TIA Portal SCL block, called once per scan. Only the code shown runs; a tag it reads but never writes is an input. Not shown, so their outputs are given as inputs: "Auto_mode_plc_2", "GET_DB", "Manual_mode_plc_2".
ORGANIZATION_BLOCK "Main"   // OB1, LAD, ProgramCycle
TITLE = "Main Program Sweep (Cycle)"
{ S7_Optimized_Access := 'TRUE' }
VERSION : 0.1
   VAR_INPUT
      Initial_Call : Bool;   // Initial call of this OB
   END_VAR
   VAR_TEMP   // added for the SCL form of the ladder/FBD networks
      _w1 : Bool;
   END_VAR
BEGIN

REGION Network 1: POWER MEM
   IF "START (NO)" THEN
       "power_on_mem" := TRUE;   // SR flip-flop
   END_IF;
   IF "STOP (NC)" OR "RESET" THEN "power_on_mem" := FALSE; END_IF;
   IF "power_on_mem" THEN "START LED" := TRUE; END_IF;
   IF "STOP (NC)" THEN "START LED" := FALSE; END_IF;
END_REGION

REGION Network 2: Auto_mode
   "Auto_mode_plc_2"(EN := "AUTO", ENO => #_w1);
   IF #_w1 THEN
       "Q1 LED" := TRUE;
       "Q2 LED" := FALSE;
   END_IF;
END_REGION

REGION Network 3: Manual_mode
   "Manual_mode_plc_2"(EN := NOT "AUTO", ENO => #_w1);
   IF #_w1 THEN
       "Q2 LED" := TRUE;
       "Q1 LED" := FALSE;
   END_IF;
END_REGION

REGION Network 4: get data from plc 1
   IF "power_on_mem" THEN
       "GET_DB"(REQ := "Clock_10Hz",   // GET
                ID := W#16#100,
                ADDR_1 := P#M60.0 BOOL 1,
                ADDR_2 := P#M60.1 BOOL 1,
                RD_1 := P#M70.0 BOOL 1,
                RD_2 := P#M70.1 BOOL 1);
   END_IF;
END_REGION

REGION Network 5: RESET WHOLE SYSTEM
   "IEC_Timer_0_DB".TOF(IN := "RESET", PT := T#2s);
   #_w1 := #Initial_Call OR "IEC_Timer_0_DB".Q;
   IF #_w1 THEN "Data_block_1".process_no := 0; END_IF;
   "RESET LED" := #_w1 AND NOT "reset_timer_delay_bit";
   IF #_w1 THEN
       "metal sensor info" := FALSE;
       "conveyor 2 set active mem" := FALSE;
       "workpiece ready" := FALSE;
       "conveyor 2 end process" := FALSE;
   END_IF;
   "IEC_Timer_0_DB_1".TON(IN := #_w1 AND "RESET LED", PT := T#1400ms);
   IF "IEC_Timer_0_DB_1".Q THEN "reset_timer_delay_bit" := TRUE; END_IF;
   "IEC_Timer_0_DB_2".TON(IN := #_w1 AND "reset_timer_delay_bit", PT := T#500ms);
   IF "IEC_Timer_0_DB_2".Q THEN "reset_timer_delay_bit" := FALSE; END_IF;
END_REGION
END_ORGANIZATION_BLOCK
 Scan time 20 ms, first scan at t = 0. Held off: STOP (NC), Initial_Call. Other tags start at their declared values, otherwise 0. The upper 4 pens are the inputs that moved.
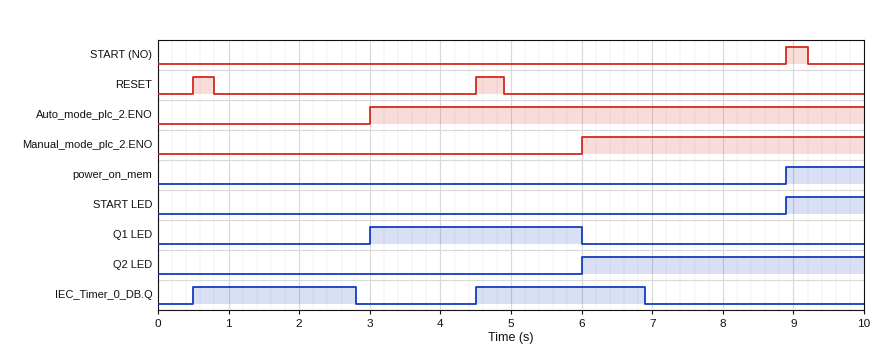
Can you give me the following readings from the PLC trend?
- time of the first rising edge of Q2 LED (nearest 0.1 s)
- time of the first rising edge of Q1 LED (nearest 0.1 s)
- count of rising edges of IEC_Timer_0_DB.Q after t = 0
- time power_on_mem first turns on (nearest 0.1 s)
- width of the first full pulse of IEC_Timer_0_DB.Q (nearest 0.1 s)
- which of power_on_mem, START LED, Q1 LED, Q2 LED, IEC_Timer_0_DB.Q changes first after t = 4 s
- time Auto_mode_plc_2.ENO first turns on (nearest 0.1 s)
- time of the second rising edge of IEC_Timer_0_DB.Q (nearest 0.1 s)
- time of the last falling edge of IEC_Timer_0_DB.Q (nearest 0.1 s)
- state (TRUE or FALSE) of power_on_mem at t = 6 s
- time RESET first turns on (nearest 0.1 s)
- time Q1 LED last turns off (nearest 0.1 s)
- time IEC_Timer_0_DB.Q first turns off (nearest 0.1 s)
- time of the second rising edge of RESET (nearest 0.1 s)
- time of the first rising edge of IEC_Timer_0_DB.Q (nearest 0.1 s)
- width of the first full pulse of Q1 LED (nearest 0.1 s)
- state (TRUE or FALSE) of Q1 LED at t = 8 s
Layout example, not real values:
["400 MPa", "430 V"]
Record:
["6.0 s", "3.0 s", "2", "8.9 s", "2.3 s", "IEC_Timer_0_DB.Q", "3.0 s", "4.5 s", "6.9 s", "FALSE", "0.5 s", "6.0 s", "2.8 s", "4.5 s", "0.5 s", "3.0 s", "FALSE"]
